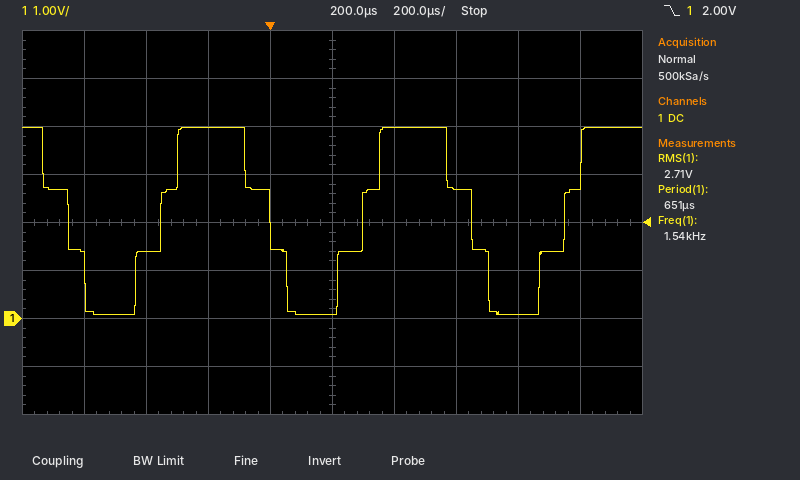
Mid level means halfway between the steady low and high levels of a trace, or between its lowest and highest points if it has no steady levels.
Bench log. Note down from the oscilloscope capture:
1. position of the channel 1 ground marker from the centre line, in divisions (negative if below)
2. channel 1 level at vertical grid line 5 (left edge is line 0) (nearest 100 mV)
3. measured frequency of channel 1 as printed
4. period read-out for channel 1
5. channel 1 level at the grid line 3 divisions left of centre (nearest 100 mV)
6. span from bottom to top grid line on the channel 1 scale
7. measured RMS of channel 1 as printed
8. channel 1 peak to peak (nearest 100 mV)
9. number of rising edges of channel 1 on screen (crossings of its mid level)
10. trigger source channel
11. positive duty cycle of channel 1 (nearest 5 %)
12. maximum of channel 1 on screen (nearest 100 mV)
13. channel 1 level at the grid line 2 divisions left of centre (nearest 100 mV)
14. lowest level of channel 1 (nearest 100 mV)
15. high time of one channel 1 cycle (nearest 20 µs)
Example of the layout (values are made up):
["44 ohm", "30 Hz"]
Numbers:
["-2.0 div", "100 mV", "1.54 kHz", "651 µs", "1.4 V", "8 V", "2.71 V", "3.9 V", "3", "channel 1", "55 %", "4.0 V", "4.0 V", "100 mV", "360 µs"]
